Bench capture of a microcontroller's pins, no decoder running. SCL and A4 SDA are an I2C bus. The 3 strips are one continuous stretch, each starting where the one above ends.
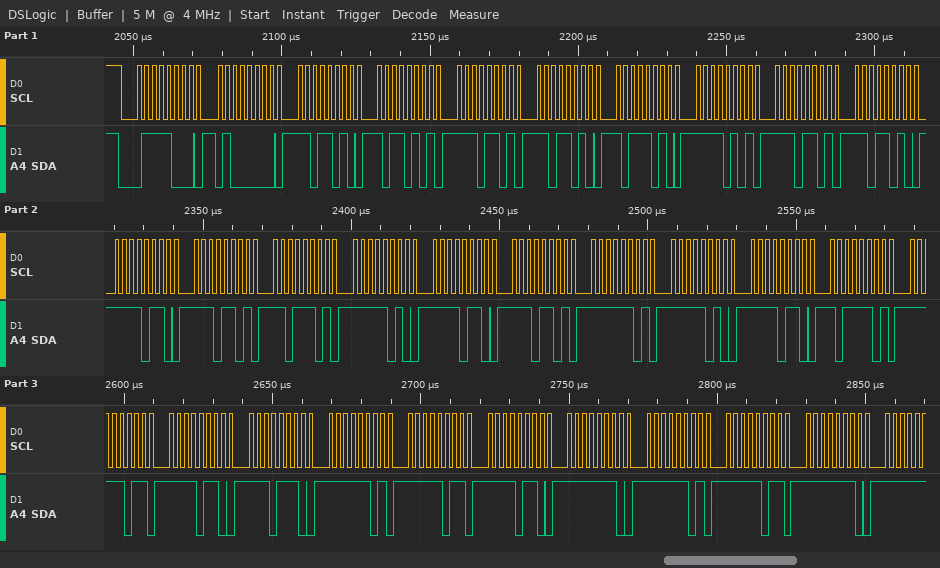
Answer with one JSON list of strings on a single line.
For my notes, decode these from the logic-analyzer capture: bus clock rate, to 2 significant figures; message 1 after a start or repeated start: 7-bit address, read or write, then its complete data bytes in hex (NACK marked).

["400 kHz", "0x3C write: 40 DA B5 ED DA BA F5 ED DA F6 ED DD FA F6 ED FD FA F6 BD FB F6 EE FD FB F6 FE FD FB FE"]
